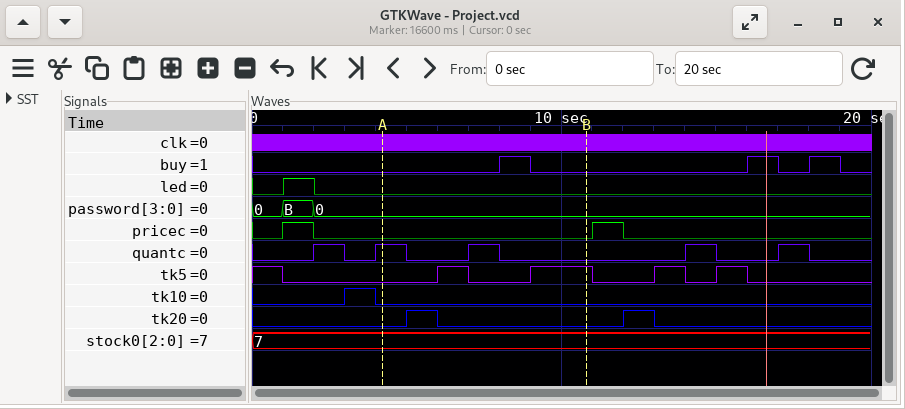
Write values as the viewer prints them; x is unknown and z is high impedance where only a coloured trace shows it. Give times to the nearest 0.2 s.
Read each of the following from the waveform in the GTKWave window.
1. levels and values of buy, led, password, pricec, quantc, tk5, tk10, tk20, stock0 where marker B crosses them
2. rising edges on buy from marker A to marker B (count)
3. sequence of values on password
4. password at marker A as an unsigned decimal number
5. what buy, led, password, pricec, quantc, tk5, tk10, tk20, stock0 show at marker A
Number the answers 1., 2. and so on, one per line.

1. buy=0, led=0, password=0, pricec=0, quantc=0, tk5=1, tk10=0, tk20=0, stock0=7
2. 1
3. 0, B, 0
4. 0
5. buy=0, led=0, password=0, pricec=0, quantc=1, tk5=0, tk10=0, tk20=0, stock0=7
